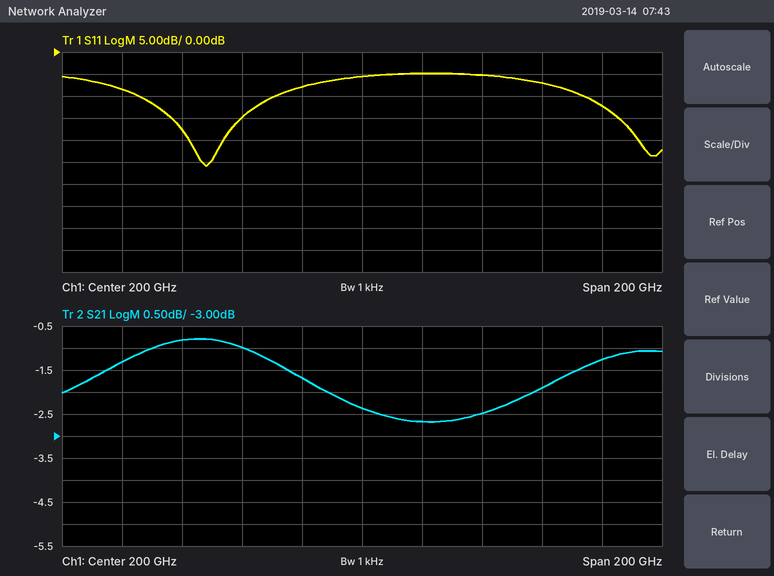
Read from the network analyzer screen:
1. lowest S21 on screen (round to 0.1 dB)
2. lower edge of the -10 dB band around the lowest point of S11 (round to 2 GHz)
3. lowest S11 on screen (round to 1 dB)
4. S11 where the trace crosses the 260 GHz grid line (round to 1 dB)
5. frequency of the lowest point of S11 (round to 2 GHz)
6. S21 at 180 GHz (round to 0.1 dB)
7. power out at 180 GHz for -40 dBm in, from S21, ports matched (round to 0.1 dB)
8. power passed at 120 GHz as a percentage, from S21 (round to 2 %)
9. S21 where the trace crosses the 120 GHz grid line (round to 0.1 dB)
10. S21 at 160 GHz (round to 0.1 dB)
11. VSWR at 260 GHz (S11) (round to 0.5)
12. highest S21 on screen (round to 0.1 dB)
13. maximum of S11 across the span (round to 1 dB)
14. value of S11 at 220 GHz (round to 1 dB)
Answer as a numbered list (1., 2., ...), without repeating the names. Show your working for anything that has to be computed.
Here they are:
1. -2.7 dB
2. 126 GHz
3. -26 dB
4. -7 dB
5. 148 GHz
6. -1.7 dB
7. -40 dBm + (-1.7 dB) = -41.7 dBm
8. 10^(-1.3/10) ≈ 74 %
9. -1.3 dB
10. -1.0 dB
11. |Γ| = 10^(-7/20) = 0.4467; VSWR = (1 + 0.4467)/(1 − 0.4467) ≈ 2.61, so 2.5 to the nearest 0.5
12. -0.8 dB
13. -5 dB
14. -5 dB
